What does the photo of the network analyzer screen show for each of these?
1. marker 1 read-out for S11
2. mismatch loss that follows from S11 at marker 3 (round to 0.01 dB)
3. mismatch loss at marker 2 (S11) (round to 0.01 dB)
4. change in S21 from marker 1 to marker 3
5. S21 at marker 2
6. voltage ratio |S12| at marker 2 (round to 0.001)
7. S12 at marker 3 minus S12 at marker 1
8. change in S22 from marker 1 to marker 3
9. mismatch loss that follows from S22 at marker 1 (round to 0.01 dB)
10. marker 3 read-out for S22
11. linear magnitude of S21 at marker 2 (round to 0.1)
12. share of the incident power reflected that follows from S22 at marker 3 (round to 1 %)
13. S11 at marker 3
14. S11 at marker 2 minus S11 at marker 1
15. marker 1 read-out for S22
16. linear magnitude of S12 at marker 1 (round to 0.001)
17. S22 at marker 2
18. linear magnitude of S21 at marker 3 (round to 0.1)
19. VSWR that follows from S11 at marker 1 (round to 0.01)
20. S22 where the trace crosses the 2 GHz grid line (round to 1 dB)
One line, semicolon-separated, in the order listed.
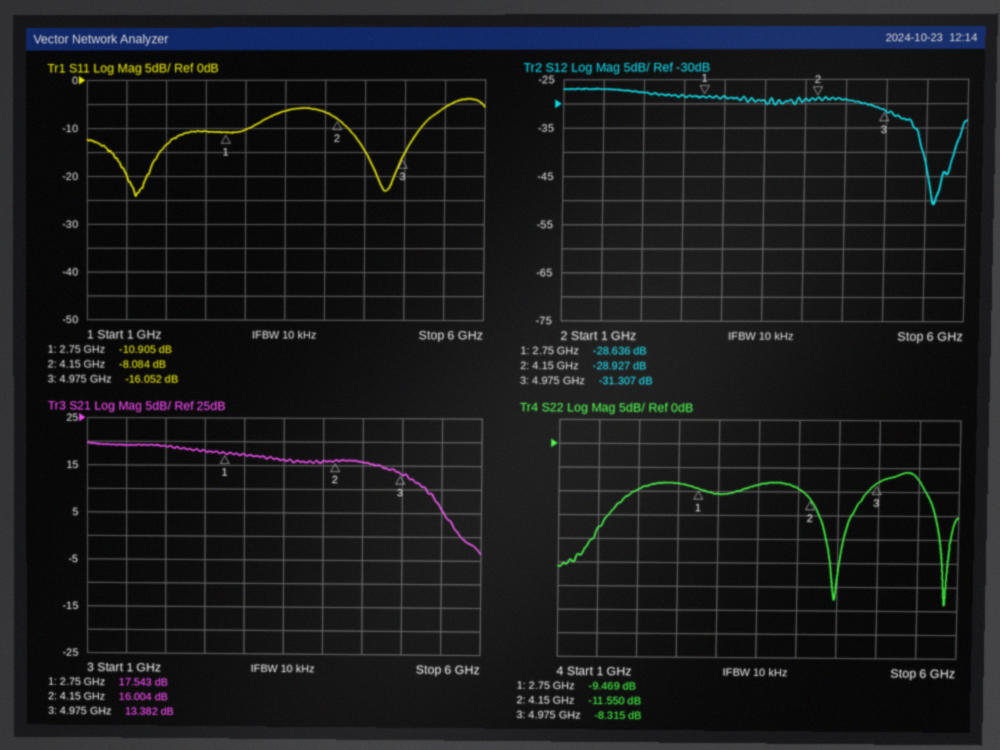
-10.905 dB; 0.11 dB; 0.73 dB; -4.161 dB; 16.004 dB; 0.036; -2.671 dB; 1.154 dB; 0.52 dB; -8.315 dB; 6.3; 15 %; -16.052 dB; 2.821 dB; -9.469 dB; 0.037; -11.550 dB; 4.7; 1.80; -10 dB
